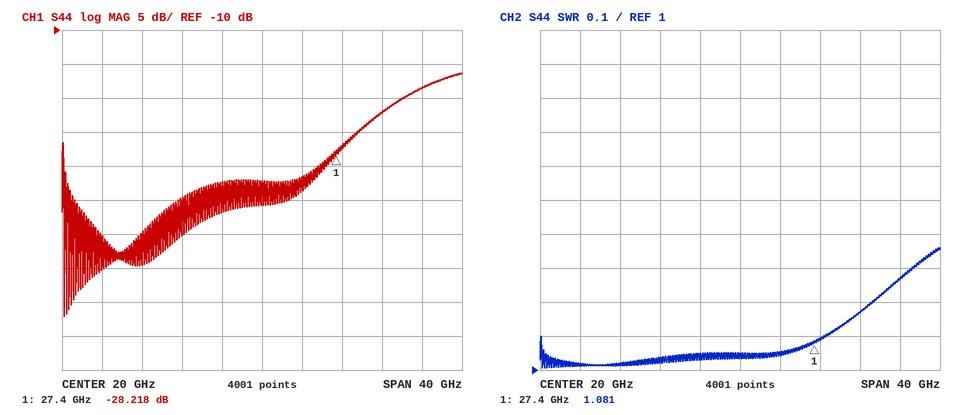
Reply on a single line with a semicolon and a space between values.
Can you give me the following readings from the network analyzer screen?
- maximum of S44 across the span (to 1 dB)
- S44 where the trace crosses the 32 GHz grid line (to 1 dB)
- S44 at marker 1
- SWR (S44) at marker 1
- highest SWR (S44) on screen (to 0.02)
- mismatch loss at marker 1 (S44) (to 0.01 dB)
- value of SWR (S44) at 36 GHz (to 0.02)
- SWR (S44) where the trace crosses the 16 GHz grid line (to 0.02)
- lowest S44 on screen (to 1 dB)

-16 dB; -22 dB; -28.218 dB; 1.081; 1.36; 0.01 dB; 1.26; 1.04; -52 dB
